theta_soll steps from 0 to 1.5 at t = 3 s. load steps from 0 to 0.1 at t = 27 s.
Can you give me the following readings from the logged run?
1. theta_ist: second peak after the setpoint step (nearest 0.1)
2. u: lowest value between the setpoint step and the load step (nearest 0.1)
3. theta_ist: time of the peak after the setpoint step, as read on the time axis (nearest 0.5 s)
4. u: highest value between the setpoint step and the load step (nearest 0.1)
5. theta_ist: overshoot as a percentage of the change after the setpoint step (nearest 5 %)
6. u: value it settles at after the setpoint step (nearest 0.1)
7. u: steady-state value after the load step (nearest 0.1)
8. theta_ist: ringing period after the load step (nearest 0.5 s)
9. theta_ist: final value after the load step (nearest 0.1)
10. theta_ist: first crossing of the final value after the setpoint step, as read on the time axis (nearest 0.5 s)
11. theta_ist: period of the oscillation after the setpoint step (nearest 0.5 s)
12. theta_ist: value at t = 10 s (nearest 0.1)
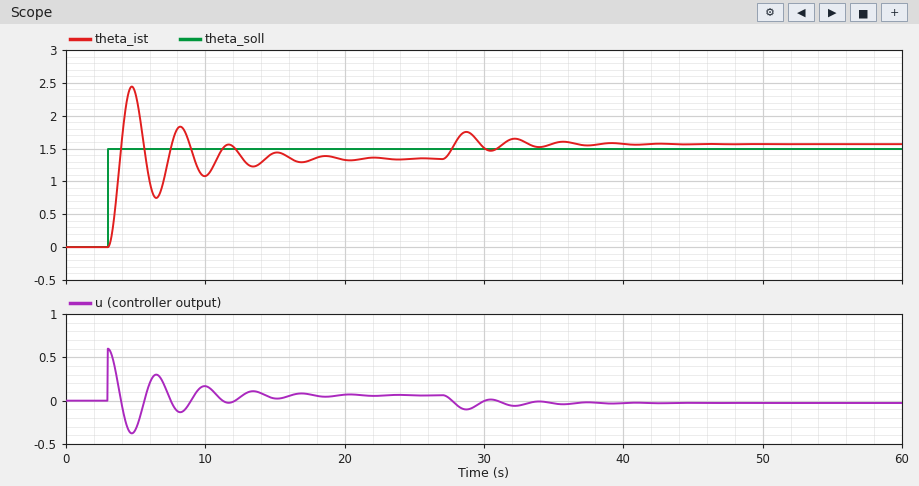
1.8
-0.4
4.5 s
0.6
80 %
0.1
0.0
3.5 s
1.6
4.0 s
3.5 s
1.1
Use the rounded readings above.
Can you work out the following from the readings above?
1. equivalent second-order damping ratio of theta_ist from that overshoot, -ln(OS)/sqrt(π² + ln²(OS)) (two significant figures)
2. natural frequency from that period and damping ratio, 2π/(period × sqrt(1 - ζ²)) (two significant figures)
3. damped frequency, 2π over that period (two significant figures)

0.071
1.8 rad/s
1.8 rad/s
